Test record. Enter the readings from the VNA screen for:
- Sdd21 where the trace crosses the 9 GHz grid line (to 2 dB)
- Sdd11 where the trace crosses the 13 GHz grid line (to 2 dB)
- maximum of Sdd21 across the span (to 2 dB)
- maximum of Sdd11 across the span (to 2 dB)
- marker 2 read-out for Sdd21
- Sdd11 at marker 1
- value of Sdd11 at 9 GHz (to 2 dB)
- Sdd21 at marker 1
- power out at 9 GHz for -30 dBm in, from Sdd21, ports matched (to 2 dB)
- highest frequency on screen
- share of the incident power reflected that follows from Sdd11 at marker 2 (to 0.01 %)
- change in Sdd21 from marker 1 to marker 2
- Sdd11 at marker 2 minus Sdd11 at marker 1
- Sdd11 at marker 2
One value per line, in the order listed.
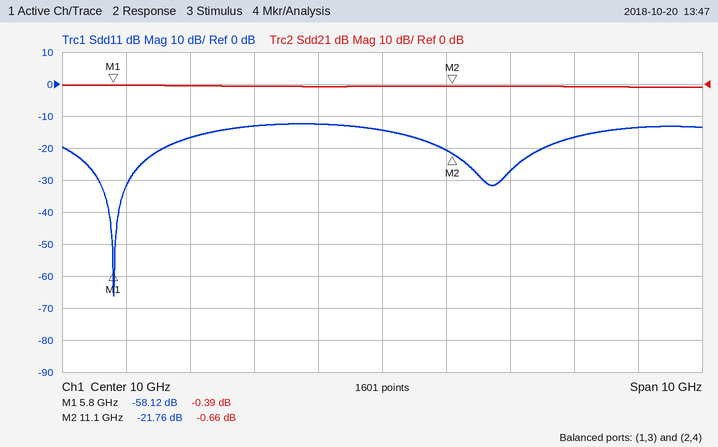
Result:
0 dB
-16 dB
0 dB
-12 dB
-0.66 dB
-58.12 dB
-12 dB
-0.39 dB
-30 dBm
15 GHz
0.67 %
-0.27 dB
36.36 dB
-21.76 dB
